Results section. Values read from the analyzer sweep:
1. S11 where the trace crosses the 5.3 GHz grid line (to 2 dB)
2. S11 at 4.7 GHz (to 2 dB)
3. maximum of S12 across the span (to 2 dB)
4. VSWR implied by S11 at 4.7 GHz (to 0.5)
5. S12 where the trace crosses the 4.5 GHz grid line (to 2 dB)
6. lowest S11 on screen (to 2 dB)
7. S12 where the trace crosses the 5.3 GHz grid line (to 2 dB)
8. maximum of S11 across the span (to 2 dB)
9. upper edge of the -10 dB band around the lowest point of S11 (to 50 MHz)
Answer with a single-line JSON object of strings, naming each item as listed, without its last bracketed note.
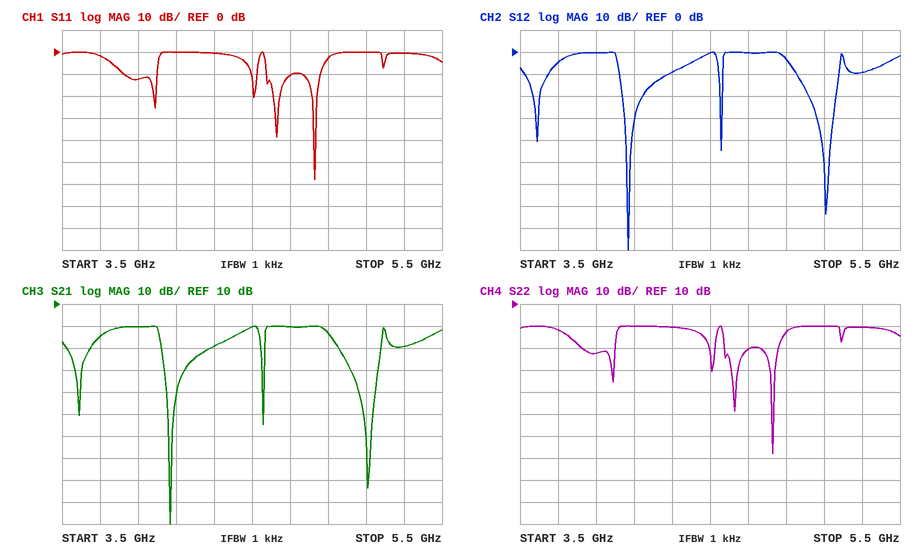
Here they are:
{"S11 where the trace crosses the 5.3 GHz grid line": "0 dB", "S11 at 4.7 GHz": "-10 dB", "maximum of S12 across the span": "0 dB", "VSWR implied by S11 at 4.7 GHz": "2.0", "S12 where the trace crosses the 4.5 GHz grid line": "0 dB", "lowest S11 on screen": "-58 dB", "S12 where the trace crosses the 5.3 GHz grid line": "-10 dB", "maximum of S11 across the span": "0 dB", "upper edge of the -10 dB band around the lowest point of S11": "4.85 GHz"}
